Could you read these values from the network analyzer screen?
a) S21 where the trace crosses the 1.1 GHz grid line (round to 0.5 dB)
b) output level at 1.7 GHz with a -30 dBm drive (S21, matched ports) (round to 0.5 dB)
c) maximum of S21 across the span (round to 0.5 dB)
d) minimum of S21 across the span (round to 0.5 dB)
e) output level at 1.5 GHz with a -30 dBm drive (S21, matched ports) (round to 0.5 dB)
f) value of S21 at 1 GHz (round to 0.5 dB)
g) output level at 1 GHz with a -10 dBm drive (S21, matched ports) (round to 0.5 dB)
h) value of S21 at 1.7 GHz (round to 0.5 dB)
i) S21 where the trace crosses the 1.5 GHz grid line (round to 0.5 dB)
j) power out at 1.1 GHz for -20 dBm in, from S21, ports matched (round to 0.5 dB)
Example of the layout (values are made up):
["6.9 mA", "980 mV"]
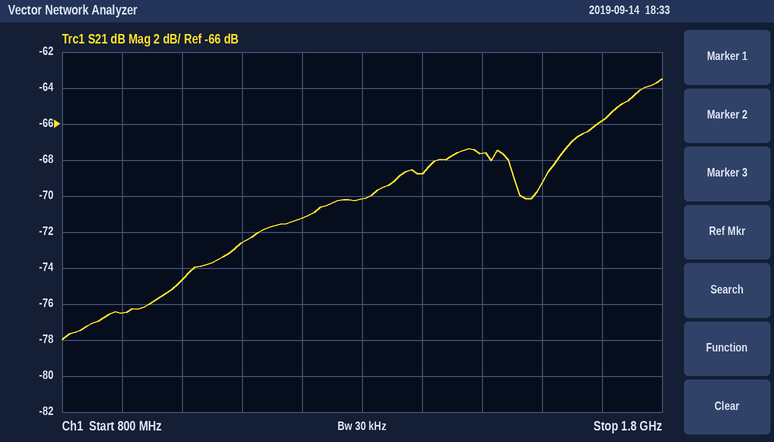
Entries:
["-72.5 dB", "-96.0 dBm", "-63.5 dB", "-78.0 dB", "-97.5 dBm", "-74.5 dB", "-84.5 dBm", "-66.0 dB", "-67.5 dB", "-92.5 dBm"]
